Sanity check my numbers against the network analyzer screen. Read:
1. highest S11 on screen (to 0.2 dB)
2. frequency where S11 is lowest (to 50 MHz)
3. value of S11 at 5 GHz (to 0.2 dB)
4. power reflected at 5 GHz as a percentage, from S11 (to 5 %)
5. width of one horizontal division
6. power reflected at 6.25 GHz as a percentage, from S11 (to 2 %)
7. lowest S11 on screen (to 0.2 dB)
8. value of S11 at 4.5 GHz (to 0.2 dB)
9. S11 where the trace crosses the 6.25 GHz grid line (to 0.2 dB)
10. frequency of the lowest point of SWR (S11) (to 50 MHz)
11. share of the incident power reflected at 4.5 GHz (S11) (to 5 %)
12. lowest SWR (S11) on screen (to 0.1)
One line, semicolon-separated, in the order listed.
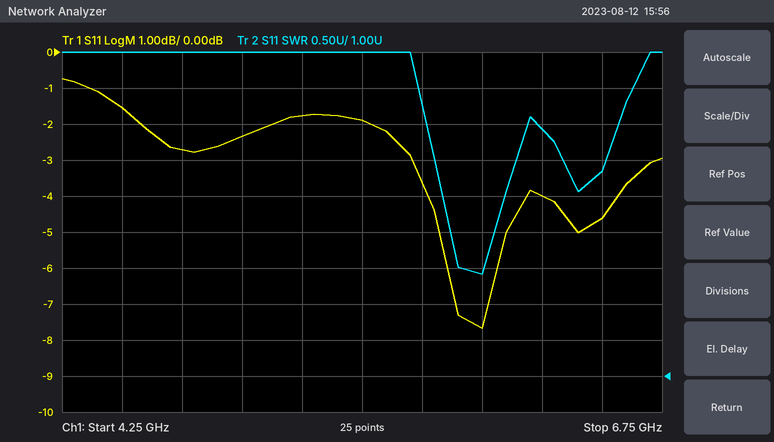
-0.8 dB; 6.00 GHz; -2.4 dB; 60 %; 250 MHz; 40 %; -7.6 dB; -1.6 dB; -4.0 dB; 6.00 GHz; 70 %; 2.4
